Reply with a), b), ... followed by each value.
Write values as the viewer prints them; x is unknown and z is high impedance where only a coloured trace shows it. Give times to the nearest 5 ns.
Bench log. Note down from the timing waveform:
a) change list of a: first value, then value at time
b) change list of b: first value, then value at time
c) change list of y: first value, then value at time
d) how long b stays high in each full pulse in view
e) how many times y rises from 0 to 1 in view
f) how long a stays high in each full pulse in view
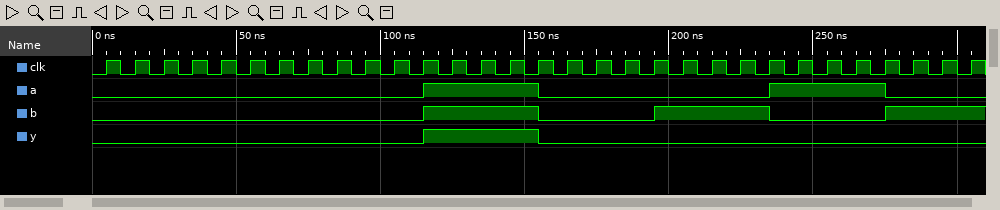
a) 0, 1 at 115 ns, 0 at 155 ns, 1 at 235 ns, 0 at 275 ns
b) 0, 1 at 115 ns, 0 at 155 ns, 1 at 195 ns, 0 at 235 ns, 1 at 275 ns
c) 0, 1 at 115 ns, 0 at 155 ns
d) 40 ns, 40 ns
e) 1
f) 40 ns, 40 ns
